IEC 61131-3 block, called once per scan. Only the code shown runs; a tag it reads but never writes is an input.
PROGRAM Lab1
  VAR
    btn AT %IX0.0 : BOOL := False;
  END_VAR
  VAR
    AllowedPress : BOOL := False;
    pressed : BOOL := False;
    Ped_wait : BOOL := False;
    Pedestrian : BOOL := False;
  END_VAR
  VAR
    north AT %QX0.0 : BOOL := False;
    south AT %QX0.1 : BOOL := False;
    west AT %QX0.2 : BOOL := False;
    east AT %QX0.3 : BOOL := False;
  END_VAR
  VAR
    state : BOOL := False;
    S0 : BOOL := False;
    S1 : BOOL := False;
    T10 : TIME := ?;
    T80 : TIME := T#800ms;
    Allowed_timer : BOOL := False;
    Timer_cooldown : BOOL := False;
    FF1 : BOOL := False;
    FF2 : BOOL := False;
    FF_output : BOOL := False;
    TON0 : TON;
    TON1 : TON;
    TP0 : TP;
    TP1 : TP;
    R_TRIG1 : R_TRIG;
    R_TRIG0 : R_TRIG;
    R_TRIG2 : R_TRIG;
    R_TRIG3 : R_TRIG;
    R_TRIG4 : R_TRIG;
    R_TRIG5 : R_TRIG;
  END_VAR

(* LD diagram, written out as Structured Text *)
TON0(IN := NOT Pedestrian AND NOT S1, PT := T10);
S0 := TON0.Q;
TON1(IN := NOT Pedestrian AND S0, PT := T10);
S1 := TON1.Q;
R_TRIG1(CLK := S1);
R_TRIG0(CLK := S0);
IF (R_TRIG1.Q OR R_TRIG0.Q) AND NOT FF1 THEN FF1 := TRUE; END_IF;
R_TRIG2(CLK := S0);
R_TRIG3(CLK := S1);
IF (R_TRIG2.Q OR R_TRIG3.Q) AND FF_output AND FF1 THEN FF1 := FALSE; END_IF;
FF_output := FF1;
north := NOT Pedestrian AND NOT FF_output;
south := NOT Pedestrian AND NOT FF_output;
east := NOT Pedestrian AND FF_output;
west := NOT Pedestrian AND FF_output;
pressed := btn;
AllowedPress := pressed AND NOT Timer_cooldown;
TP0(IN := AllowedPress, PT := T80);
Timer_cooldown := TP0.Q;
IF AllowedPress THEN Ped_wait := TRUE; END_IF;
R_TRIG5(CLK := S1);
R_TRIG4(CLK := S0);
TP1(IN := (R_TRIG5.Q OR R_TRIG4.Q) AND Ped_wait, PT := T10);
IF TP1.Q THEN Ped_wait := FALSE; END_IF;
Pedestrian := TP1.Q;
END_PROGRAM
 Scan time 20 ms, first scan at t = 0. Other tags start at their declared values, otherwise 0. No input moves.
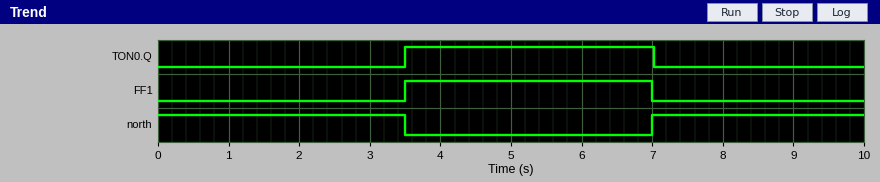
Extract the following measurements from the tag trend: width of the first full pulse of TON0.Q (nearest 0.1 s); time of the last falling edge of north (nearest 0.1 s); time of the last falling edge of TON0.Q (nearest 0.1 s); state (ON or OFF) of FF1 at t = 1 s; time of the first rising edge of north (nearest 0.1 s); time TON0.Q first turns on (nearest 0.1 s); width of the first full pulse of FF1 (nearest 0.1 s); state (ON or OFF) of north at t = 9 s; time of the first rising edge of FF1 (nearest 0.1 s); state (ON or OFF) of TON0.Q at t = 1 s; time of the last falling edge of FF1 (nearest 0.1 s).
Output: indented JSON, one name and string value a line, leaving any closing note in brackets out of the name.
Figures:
{
  "width of the first full pulse of TON0.Q": "3.5 s",
  "time of the last falling edge of north": "3.5 s",
  "time of the last falling edge of TON0.Q": "7.0 s",
  "state (ON or OFF) of FF1 at t = 1 s": "OFF",
  "time of the first rising edge of north": "7.0 s",
  "time TON0.Q first turns on": "3.5 s",
  "width of the first full pulse of FF1": "3.5 s",
  "state (ON or OFF) of north at t = 9 s": "ON",
  "time of the first rising edge of FF1": "3.5 s",
  "state (ON or OFF) of TON0.Q at t = 1 s": "OFF",
  "time of the last falling edge of FF1": "7.0 s"
}
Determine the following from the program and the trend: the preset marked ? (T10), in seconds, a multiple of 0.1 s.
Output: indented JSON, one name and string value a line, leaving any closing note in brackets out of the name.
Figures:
{
  "the preset marked ? (T10), in seconds, a multiple of 0.1 s": "3.5 s"
}
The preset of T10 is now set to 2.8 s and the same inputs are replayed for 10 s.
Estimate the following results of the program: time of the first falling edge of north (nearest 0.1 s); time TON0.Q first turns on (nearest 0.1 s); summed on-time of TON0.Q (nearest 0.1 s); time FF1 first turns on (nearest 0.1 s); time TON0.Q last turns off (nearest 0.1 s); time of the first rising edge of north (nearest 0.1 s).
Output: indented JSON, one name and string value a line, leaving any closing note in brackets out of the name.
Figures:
{
  "time of the first falling edge of north": "2.8 s",
  "time TON0.Q first turns on": "2.8 s",
  "summed on-time of TON0.Q": "4.4 s",
  "time FF1 first turns on": "2.8 s",
  "time TON0.Q last turns off": "5.6 s",
  "time of the first rising edge of north": "5.6 s"
}
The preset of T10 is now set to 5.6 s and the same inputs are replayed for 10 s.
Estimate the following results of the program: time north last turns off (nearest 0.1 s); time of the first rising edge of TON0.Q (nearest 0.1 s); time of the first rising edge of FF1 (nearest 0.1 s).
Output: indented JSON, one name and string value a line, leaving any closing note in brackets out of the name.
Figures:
{
  "time north last turns off": "5.6 s",
  "time of the first rising edge of TON0.Q": "5.6 s",
  "time of the first rising edge of FF1": "5.6 s"
}
